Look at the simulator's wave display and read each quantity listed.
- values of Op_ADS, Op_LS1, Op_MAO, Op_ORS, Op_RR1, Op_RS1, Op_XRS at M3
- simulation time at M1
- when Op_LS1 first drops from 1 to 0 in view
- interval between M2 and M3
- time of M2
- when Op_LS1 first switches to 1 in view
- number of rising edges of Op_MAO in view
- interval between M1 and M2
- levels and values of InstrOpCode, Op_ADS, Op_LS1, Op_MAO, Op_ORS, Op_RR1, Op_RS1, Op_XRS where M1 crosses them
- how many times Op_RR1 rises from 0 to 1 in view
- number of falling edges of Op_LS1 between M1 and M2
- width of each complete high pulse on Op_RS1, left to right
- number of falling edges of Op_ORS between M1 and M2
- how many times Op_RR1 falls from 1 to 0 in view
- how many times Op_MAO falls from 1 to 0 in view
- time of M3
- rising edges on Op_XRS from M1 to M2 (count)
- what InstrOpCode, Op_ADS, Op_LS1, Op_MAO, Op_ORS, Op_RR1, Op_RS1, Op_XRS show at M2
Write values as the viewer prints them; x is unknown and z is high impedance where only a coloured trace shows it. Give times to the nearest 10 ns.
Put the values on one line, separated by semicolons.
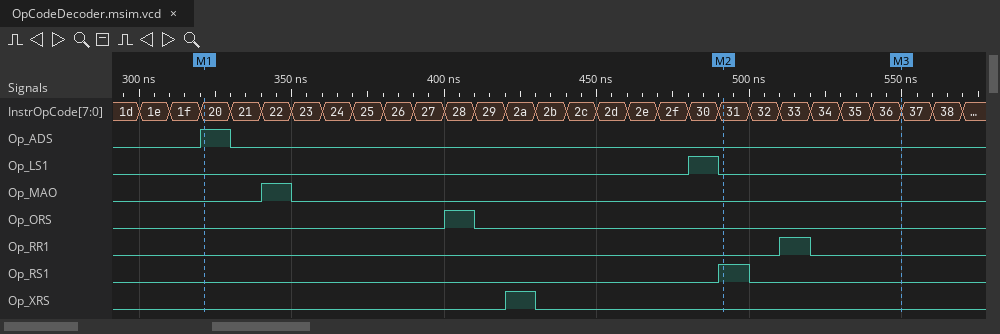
Op_ADS=0, Op_LS1=0, Op_MAO=0, Op_ORS=0, Op_RR1=0, Op_RS1=0, Op_XRS=0; 320 ns; 490 ns; 60 ns; 490 ns; 480 ns; 1; 170 ns; InstrOpCode=20, Op_ADS=1, Op_LS1=0, Op_MAO=0, Op_ORS=0, Op_RR1=0, Op_RS1=0, Op_XRS=0; 1; 1; 10 ns; 1; 1; 1; 550 ns; 1; InstrOpCode=31, Op_ADS=0, Op_LS1=0, Op_MAO=0, Op_ORS=0, Op_RR1=0, Op_RS1=1, Op_XRS=0
